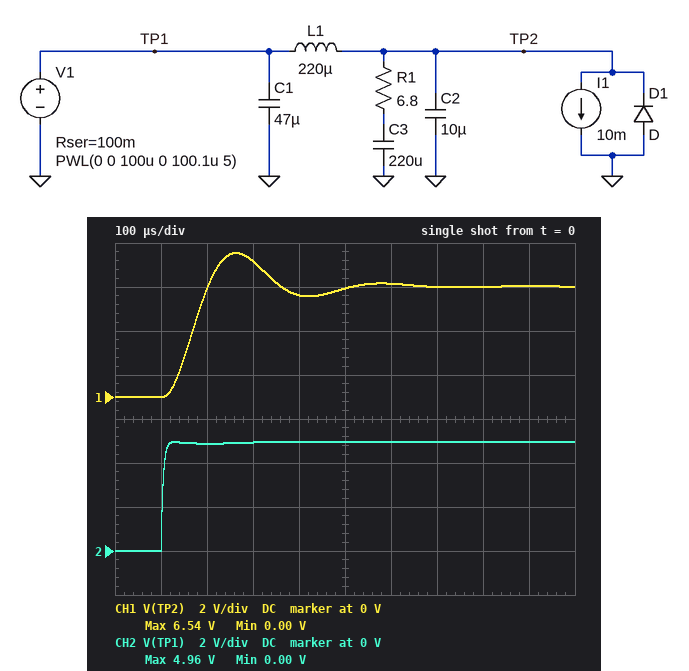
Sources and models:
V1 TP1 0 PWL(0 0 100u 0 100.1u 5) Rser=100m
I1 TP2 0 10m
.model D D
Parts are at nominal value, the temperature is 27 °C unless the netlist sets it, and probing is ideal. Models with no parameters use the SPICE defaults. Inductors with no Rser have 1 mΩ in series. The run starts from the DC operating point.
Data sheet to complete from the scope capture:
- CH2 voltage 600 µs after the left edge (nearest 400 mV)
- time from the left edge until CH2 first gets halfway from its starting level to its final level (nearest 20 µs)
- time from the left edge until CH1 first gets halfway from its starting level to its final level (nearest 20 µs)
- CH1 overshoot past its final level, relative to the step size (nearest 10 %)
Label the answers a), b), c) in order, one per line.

a) 4.8 V
b) 100 µs
c) 160 µs
d) 30 %
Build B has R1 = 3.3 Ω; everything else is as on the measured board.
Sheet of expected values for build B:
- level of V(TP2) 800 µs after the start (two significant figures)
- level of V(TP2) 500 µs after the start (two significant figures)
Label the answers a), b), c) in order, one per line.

a) 5.1 V
b) 5.2 V
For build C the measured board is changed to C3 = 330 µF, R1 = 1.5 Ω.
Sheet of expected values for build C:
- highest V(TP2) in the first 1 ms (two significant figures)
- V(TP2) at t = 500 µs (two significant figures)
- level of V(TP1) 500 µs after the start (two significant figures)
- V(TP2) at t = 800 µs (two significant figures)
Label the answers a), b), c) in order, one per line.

a) 5.6 V
b) 5.4 V
c) 4.8 V
d) 5.5 V
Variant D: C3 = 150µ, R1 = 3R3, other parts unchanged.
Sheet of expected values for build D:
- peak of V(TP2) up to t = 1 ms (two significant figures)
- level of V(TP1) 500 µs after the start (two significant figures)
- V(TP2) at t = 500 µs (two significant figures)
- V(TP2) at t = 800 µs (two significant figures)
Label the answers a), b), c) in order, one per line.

a) 5.6 V
b) 4.9 V
c) 5.3 V
d) 5.2 V
